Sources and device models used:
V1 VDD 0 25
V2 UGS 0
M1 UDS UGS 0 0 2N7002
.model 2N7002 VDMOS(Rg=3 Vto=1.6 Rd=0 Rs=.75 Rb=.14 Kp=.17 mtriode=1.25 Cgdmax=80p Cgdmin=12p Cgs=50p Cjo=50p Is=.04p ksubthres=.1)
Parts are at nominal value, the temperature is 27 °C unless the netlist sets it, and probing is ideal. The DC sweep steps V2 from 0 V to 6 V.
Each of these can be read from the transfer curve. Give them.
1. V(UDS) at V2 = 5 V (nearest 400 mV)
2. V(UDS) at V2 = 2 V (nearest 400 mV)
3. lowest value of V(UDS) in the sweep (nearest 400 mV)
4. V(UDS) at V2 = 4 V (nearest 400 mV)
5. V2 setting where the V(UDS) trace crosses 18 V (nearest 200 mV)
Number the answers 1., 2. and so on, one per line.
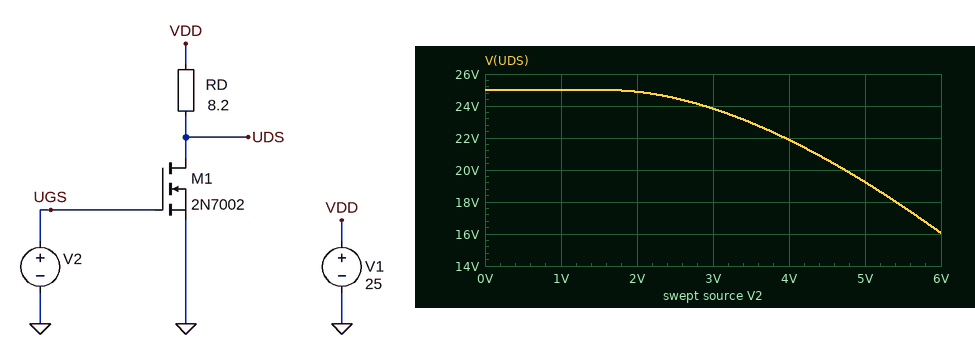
1. 19.2 V
2. 24.8 V
3. 16.0 V
4. 22.0 V
5. 5.4 V
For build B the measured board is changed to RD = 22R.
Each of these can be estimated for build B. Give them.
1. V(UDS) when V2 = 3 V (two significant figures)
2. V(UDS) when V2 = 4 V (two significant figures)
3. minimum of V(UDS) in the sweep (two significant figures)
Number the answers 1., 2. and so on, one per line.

1. 22 V
2. 17 V
3. 2.7 V
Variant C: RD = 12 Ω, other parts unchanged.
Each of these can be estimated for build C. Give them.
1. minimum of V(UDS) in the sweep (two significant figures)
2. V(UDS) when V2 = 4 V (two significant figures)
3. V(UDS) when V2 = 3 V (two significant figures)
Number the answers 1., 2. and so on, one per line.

1. 12 V
2. 20 V
3. 23 V
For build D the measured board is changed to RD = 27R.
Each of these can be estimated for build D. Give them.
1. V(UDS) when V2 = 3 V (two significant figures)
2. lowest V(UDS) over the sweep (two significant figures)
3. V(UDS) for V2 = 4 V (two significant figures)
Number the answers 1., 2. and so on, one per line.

1. 21 V
2. 2.0 V
3. 15 V
